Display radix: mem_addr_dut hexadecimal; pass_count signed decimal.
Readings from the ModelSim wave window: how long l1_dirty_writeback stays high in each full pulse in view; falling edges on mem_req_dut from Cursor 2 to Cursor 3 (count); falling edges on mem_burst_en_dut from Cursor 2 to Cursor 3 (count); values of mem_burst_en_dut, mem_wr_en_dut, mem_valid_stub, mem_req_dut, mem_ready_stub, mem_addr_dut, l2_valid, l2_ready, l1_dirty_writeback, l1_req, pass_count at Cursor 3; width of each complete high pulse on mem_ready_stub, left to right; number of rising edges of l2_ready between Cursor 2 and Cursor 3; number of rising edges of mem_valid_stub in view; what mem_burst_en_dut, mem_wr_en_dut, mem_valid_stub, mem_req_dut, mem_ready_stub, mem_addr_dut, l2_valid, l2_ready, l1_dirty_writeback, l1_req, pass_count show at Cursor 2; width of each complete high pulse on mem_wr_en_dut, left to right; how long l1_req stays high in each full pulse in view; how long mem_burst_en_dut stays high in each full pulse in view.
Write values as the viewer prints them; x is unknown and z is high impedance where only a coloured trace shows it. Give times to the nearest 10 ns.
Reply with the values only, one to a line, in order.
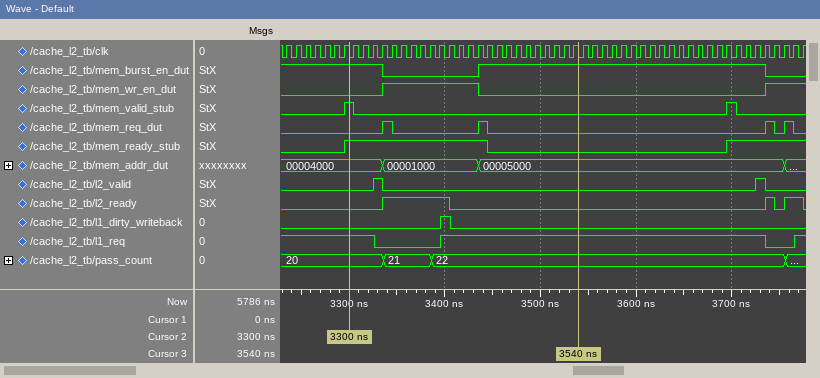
10 ns
2
1
mem_burst_en_dut=1, mem_wr_en_dut=0, mem_valid_stub=0, mem_req_dut=0, mem_ready_stub=0, mem_addr_dut=00005000, l2_valid=0, l2_ready=0, l1_dirty_writeback=0, l1_req=1, pass_count=22
150 ns
1
2
mem_burst_en_dut=1, mem_wr_en_dut=0, mem_valid_stub=1, mem_req_dut=0, mem_ready_stub=1, mem_addr_dut=00004000, l2_valid=0, l2_ready=0, l1_dirty_writeback=0, l1_req=1, pass_count=20
100 ns
340 ns
300 ns
